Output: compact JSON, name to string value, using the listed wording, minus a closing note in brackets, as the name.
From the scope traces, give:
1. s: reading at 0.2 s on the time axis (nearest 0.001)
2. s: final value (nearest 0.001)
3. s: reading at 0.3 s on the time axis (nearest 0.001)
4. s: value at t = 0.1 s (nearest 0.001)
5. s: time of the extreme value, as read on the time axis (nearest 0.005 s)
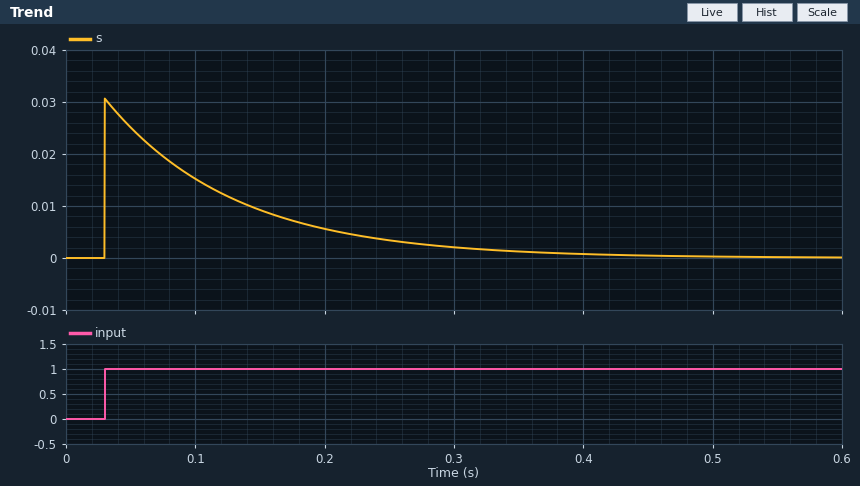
{"s: reading at 0.2 s on the time axis": "0.006", "s: final value": "0.000", "s: reading at 0.3 s on the time axis": "0.002", "s: value at t = 0.1 s": "0.015", "s: time of the extreme value, as read on the time axis": "0.030 s"}
